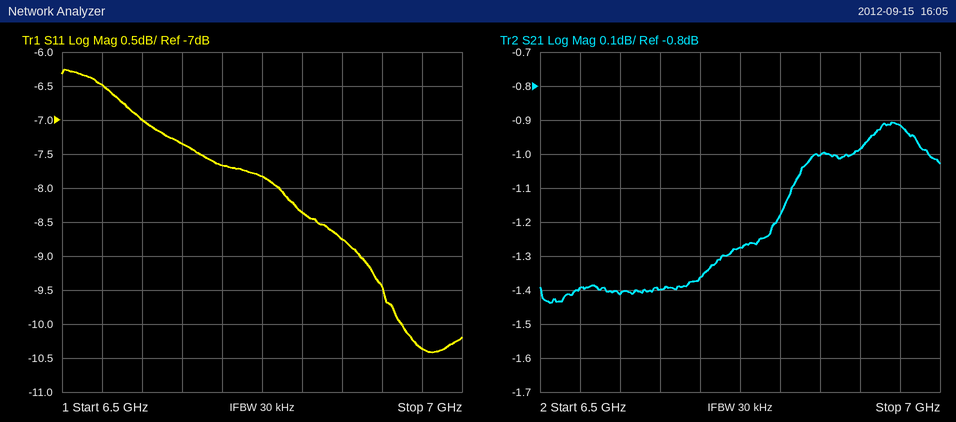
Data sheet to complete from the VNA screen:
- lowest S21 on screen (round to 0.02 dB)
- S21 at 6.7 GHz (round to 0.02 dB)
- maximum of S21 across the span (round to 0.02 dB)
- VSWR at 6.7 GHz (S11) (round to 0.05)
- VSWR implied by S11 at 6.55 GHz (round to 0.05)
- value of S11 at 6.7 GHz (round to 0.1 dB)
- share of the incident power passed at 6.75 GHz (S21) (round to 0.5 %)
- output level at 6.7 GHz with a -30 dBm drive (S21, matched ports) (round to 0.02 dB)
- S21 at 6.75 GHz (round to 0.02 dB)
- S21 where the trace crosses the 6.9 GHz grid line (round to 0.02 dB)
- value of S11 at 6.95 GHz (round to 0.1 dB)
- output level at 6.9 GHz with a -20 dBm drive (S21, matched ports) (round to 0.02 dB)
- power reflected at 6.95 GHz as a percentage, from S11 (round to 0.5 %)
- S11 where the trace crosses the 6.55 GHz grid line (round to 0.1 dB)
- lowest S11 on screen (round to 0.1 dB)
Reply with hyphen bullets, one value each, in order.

- -1.44 dB
- -1.36 dB
- -0.90 dB
- 2.40
- 2.80
- -7.7 dB
- 74.5 %
- -31.36 dBm
- -1.28 dB
- -0.98 dB
- -10.4 dB
- -20.98 dBm
- 9.0 %
- -6.5 dB
- -10.4 dB
